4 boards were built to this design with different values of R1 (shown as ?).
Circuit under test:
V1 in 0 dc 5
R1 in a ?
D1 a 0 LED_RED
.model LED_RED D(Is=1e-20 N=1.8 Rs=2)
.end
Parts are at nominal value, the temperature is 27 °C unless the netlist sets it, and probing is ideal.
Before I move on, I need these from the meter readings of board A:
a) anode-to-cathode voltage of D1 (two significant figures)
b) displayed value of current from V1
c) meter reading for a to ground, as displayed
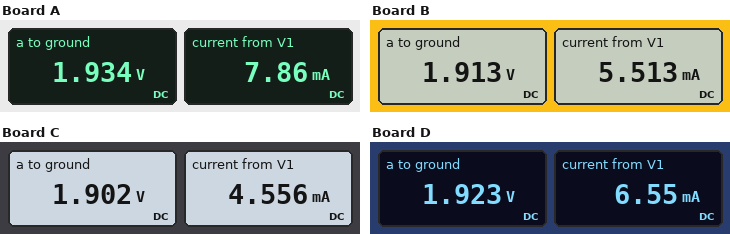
1.9 V
7.86 mA
1.934 V
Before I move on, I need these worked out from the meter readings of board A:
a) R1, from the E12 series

390 Ω
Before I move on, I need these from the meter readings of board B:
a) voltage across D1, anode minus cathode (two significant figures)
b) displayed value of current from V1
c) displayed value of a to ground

1.9 V
5.513 mA
1.913 V
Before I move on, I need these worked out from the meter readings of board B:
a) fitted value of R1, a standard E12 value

560 Ω
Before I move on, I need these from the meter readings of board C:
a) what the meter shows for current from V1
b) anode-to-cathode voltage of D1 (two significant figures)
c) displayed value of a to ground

4.556 mA
1.9 V
1.902 V
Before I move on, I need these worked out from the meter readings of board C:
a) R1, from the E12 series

680 Ω
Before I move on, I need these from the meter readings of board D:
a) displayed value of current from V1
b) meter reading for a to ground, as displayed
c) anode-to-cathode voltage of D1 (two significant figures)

6.55 mA
1.923 V
1.9 V
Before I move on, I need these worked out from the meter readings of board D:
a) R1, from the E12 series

470 Ω
